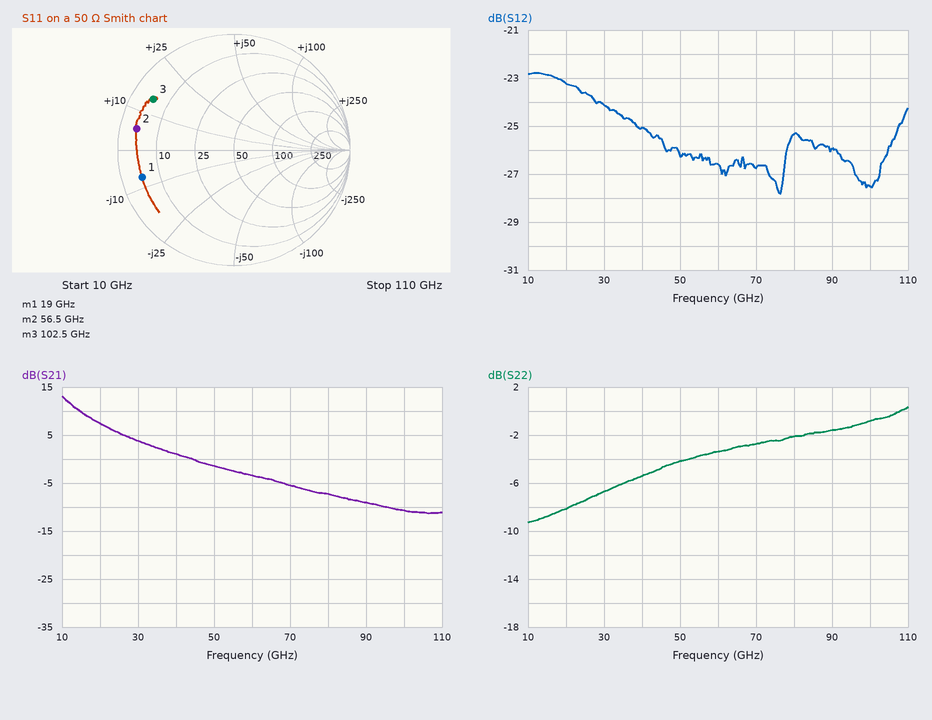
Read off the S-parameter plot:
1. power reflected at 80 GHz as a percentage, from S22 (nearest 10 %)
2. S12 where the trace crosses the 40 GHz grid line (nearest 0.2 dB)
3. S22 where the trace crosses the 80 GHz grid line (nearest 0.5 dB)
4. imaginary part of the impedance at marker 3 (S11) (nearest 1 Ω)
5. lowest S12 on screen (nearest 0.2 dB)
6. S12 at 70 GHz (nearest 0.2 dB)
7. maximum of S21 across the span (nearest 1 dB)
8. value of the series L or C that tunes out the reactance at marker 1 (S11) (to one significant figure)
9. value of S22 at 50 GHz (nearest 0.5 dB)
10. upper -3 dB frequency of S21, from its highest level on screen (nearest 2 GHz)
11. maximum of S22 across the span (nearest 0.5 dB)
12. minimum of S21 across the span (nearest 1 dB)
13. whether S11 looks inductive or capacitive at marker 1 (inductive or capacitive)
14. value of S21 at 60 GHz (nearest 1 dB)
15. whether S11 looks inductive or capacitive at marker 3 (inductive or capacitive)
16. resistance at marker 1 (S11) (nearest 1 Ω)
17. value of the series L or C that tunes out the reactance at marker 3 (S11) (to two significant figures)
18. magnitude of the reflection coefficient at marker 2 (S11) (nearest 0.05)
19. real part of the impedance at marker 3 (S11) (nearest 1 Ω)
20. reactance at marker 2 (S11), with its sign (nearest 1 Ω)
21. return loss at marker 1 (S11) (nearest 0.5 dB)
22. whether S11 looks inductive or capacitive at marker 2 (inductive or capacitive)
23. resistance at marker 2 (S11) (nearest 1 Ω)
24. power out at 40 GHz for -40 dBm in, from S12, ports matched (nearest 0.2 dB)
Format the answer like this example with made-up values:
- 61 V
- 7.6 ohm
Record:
- 60 %
- -25.0 dB
- -2.0 dB
- +14 Ω
- -27.8 dB
- -26.8 dB
- 13 dB
- 60 pH
- -4.0 dB
- 14 GHz
- 0.5 dB
- -11 dB
- capacitive
- -3 dB
- inductive
- 5 Ω
- 110 fF
- 0.85
- 5 Ω
- +5 Ω
- 1.5 dB
- inductive
- 4 Ω
- -65.0 dBm
